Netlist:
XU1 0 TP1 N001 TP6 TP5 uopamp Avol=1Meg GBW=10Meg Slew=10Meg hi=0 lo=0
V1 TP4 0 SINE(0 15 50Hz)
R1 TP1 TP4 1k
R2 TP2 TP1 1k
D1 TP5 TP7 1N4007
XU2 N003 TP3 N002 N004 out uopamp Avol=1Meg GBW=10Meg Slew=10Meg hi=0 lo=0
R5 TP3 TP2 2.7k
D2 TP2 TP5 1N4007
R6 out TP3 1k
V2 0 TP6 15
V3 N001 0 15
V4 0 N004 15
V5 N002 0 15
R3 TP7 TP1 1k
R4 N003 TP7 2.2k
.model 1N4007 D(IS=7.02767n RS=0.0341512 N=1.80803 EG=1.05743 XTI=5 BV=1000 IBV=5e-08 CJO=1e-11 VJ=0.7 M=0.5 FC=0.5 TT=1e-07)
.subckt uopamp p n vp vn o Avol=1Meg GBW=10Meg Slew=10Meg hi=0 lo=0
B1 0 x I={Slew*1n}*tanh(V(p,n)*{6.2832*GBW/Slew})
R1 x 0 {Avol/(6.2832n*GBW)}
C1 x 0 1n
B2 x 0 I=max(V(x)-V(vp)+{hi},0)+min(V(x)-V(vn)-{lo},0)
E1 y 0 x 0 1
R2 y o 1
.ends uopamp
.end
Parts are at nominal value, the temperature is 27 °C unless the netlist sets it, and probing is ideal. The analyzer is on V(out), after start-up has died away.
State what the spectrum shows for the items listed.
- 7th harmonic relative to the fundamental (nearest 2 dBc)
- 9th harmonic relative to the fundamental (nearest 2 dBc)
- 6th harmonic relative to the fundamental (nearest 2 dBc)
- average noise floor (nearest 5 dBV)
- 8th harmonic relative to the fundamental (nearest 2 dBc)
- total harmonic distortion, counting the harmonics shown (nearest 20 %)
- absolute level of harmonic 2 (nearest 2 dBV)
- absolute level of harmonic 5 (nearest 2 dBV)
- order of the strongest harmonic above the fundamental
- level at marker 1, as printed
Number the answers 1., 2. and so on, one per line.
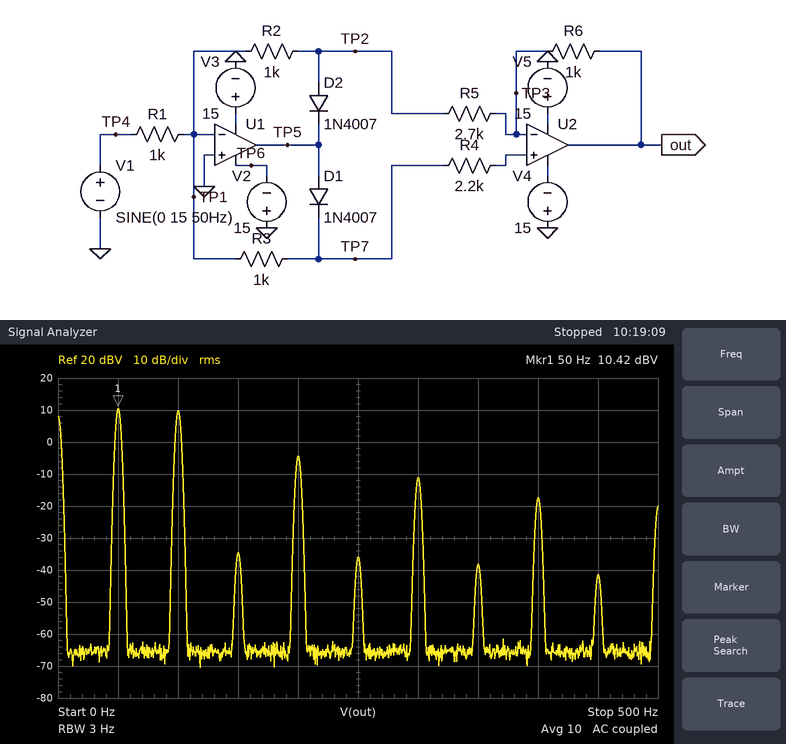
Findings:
1. -48 dBc
2. -52 dBc
3. -22 dBc
4. -65 dBV
5. -28 dBc
6. 100 %
7. 10 dBV
8. -36 dBV
9. 2
10. 10.42 dBV
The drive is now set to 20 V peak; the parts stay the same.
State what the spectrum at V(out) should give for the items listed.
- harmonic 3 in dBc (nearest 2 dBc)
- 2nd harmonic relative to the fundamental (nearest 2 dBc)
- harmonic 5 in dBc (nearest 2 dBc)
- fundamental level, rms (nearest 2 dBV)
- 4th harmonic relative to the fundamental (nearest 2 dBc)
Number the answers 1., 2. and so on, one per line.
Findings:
1. -10 dBc
2. 2 dBc
3. -22 dBc
4. 10 dBV
5. -8 dBc
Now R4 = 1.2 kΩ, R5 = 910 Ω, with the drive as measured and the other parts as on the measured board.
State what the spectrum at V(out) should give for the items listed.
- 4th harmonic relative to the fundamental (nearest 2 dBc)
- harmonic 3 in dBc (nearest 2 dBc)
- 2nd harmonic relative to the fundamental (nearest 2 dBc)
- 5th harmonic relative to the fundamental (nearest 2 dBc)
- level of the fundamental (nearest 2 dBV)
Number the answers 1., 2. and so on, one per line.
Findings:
1. 10 dBc
2. -6 dBc
3. 22 dBc
4. -10 dBc
5. -10 dBV
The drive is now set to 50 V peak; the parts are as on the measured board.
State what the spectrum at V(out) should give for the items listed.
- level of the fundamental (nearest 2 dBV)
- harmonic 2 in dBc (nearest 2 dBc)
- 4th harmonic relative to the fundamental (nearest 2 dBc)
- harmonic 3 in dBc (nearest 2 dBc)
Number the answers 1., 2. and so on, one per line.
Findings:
1. -8 dBV
2. 18 dBc
3. 16 dBc
4. 8 dBc
